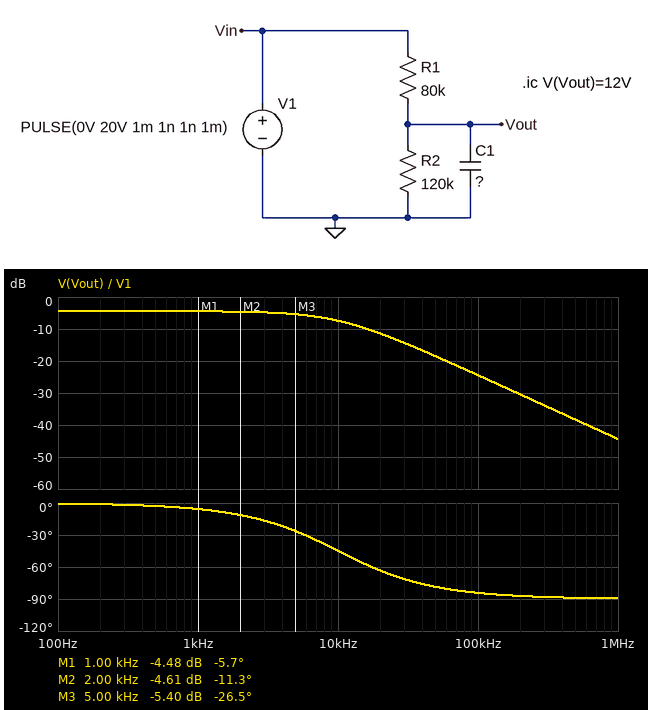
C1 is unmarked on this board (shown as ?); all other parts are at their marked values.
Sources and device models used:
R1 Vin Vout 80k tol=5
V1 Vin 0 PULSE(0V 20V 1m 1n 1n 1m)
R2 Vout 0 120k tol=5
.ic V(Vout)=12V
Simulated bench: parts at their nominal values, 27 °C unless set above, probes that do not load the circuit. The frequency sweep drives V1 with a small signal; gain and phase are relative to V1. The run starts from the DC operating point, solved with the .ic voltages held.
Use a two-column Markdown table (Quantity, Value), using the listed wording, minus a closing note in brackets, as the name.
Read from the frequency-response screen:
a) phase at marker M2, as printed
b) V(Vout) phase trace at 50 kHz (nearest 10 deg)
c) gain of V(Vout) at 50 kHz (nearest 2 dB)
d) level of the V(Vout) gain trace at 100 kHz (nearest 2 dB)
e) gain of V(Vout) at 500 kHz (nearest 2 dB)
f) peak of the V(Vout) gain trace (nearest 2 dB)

| Quantity | Value |
|---|---|
| phase at marker M2, as printed | -11.3 deg |
| V(Vout) phase trace at 50 kHz | -80 deg |
| gain of V(Vout) at 50 kHz | -18 dB |
| level of the V(Vout) gain trace at 100 kHz | -24 dB |
| gain of V(Vout) at 500 kHz | -38 dB |
| peak of the V(Vout) gain trace | -4 dB |
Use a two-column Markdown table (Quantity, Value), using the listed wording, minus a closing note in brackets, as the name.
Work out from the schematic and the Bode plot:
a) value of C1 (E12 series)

| Quantity | Value |
|---|---|
| value of C1 | 330 pF |
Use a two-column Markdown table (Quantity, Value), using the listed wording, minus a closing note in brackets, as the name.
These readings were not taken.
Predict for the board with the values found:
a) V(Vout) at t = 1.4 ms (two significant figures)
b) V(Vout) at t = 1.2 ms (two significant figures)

| Quantity | Value |
|---|---|
| V(Vout) at t = 1.4 ms | 12 V |
| V(Vout) at t = 1.2 ms | 12 V |
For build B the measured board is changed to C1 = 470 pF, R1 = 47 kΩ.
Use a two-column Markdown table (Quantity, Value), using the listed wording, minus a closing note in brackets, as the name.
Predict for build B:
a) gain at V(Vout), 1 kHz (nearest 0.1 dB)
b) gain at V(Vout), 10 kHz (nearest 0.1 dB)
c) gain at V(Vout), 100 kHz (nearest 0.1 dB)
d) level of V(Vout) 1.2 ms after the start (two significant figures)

| Quantity | Value |
|---|---|
| gain at V(Vout), 1 kHz | -2.9 dB |
| gain at V(Vout), 10 kHz | -5.9 dB |
| gain at V(Vout), 100 kHz | -22.9 dB |
| level of V(Vout) 1.2 ms after the start | 14 V |
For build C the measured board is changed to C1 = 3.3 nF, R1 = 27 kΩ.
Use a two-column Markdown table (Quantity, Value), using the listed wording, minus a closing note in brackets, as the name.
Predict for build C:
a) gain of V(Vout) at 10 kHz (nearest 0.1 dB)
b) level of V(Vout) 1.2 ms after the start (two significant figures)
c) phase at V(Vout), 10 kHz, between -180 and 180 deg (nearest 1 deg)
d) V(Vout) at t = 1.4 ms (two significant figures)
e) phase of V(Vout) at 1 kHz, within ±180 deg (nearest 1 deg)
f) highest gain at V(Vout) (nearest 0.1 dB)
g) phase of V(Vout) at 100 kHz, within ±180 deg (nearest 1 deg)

| Quantity | Value |
|---|---|
| gain of V(Vout) at 10 kHz | -15.2 dB |
| level of V(Vout) 1.2 ms after the start | 15 V |
| phase at V(Vout), 10 kHz, between -180 and 180 deg | -78 deg |
| V(Vout) at t = 1.4 ms | 16 V |
| phase of V(Vout) at 1 kHz, within ±180 deg | -25 deg |
| highest gain at V(Vout) | -1.8 dB |
| phase of V(Vout) at 100 kHz, within ±180 deg | -89 deg |
